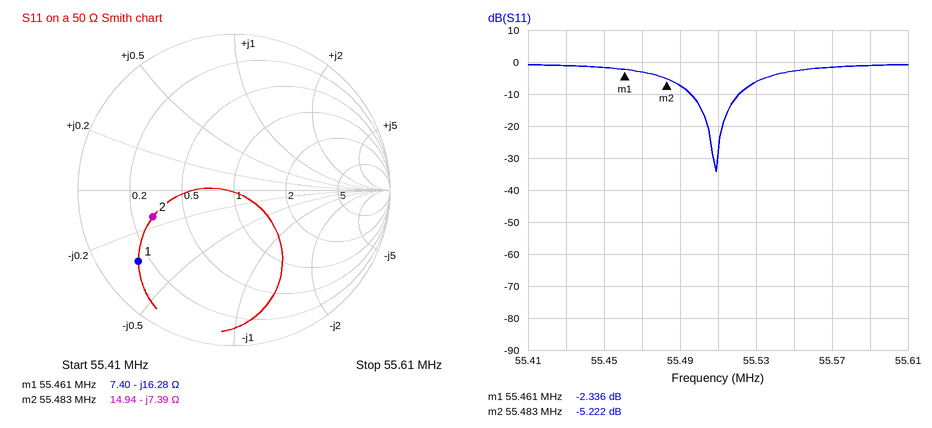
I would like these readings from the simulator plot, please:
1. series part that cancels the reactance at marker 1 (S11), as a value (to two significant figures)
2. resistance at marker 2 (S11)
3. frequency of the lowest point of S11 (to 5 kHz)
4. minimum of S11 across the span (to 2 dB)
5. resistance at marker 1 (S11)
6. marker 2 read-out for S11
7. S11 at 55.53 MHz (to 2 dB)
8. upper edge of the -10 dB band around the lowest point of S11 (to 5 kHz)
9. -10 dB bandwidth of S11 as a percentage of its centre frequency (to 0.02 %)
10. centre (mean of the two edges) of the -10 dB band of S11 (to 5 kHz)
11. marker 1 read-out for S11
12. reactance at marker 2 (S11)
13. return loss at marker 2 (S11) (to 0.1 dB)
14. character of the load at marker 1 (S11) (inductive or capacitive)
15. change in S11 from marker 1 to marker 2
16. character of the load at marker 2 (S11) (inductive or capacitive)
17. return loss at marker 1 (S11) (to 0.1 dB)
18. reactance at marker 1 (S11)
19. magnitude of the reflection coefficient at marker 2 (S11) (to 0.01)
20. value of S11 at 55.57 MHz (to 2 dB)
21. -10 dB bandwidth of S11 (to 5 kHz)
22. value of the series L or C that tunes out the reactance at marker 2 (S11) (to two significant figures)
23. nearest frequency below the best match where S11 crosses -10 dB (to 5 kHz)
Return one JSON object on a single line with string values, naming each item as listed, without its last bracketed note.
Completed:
{"series part that cancels the reactance at marker 1 (S11), as a value": "47 nH", "resistance at marker 2": "14.94 Ω", "frequency of the lowest point of S11": "55.510 MHz", "minimum of S11 across the span": "-34 dB", "resistance at marker 1": "7.40 Ω", "marker 2 read-out for S11": "-5.222 dB", "S11 at 55.53 MHz": "-6 dB", "upper edge of the -10 dB band around the lowest point of S11": "55.520 MHz", "-10 dB bandwidth of S11 as a percentage of its centre frequency": "0.04 %", "centre (mean of the two edges) of the -10 dB band of S11": "55.510 MHz", "marker 1 read-out for S11": "-2.336 dB", "reactance at marker 2": "-7.39 Ω", "return loss at marker 2 (S11)": "5.2 dB", "character of the load at marker 1 (S11)": "capacitive", "change in S11 from marker 1 to marker 2": "-2.886 dB", "character of the load at marker 2 (S11)": "capacitive", "return loss at marker 1 (S11)": "2.3 dB", "reactance at marker 1": "-16.28 Ω", "magnitude of the reflection coefficient at marker 2 (S11)": "0.55", "value of S11 at 55.57 MHz": "-2 dB", "-10 dB bandwidth of S11": "25 kHz", "value of the series L or C that tunes out the reactance at marker 2 (S11)": "21 nH", "nearest frequency below the best match where S11 crosses -10 dB": "55.495 MHz"}
